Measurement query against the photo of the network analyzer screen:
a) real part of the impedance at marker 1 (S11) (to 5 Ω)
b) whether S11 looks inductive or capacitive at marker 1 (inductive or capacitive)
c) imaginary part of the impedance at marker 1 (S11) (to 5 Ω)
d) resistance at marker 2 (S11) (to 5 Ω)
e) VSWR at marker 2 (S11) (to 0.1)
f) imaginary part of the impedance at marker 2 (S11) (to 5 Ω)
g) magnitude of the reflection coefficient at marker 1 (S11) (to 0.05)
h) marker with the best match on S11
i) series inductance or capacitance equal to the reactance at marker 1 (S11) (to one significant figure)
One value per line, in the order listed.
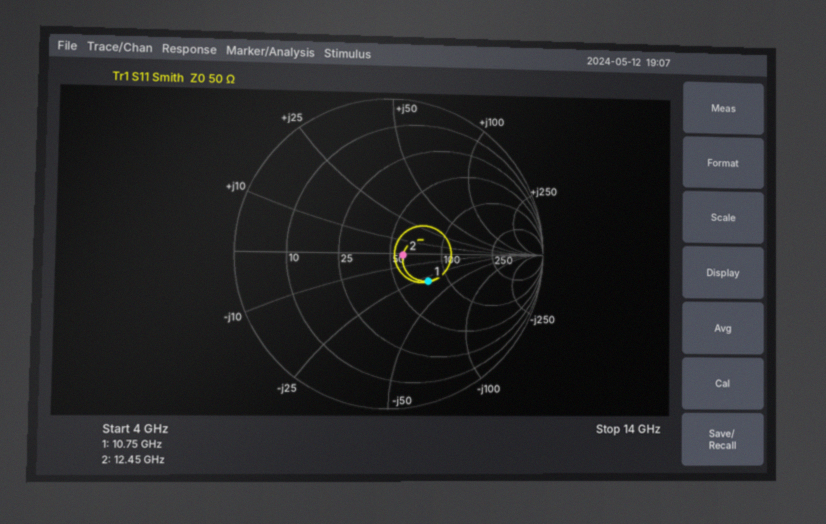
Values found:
75 Ω
capacitive
-30 Ω
60 Ω
1.2
0 Ω
0.30
marker 2
500 fF
